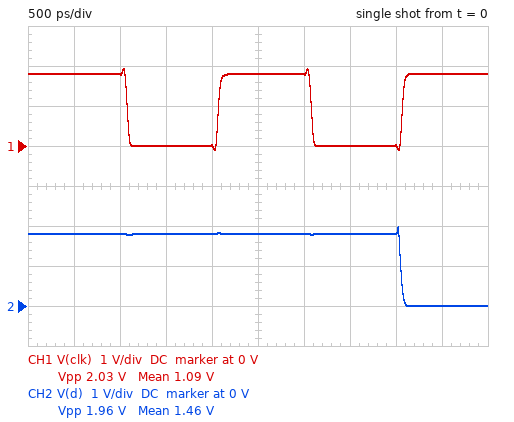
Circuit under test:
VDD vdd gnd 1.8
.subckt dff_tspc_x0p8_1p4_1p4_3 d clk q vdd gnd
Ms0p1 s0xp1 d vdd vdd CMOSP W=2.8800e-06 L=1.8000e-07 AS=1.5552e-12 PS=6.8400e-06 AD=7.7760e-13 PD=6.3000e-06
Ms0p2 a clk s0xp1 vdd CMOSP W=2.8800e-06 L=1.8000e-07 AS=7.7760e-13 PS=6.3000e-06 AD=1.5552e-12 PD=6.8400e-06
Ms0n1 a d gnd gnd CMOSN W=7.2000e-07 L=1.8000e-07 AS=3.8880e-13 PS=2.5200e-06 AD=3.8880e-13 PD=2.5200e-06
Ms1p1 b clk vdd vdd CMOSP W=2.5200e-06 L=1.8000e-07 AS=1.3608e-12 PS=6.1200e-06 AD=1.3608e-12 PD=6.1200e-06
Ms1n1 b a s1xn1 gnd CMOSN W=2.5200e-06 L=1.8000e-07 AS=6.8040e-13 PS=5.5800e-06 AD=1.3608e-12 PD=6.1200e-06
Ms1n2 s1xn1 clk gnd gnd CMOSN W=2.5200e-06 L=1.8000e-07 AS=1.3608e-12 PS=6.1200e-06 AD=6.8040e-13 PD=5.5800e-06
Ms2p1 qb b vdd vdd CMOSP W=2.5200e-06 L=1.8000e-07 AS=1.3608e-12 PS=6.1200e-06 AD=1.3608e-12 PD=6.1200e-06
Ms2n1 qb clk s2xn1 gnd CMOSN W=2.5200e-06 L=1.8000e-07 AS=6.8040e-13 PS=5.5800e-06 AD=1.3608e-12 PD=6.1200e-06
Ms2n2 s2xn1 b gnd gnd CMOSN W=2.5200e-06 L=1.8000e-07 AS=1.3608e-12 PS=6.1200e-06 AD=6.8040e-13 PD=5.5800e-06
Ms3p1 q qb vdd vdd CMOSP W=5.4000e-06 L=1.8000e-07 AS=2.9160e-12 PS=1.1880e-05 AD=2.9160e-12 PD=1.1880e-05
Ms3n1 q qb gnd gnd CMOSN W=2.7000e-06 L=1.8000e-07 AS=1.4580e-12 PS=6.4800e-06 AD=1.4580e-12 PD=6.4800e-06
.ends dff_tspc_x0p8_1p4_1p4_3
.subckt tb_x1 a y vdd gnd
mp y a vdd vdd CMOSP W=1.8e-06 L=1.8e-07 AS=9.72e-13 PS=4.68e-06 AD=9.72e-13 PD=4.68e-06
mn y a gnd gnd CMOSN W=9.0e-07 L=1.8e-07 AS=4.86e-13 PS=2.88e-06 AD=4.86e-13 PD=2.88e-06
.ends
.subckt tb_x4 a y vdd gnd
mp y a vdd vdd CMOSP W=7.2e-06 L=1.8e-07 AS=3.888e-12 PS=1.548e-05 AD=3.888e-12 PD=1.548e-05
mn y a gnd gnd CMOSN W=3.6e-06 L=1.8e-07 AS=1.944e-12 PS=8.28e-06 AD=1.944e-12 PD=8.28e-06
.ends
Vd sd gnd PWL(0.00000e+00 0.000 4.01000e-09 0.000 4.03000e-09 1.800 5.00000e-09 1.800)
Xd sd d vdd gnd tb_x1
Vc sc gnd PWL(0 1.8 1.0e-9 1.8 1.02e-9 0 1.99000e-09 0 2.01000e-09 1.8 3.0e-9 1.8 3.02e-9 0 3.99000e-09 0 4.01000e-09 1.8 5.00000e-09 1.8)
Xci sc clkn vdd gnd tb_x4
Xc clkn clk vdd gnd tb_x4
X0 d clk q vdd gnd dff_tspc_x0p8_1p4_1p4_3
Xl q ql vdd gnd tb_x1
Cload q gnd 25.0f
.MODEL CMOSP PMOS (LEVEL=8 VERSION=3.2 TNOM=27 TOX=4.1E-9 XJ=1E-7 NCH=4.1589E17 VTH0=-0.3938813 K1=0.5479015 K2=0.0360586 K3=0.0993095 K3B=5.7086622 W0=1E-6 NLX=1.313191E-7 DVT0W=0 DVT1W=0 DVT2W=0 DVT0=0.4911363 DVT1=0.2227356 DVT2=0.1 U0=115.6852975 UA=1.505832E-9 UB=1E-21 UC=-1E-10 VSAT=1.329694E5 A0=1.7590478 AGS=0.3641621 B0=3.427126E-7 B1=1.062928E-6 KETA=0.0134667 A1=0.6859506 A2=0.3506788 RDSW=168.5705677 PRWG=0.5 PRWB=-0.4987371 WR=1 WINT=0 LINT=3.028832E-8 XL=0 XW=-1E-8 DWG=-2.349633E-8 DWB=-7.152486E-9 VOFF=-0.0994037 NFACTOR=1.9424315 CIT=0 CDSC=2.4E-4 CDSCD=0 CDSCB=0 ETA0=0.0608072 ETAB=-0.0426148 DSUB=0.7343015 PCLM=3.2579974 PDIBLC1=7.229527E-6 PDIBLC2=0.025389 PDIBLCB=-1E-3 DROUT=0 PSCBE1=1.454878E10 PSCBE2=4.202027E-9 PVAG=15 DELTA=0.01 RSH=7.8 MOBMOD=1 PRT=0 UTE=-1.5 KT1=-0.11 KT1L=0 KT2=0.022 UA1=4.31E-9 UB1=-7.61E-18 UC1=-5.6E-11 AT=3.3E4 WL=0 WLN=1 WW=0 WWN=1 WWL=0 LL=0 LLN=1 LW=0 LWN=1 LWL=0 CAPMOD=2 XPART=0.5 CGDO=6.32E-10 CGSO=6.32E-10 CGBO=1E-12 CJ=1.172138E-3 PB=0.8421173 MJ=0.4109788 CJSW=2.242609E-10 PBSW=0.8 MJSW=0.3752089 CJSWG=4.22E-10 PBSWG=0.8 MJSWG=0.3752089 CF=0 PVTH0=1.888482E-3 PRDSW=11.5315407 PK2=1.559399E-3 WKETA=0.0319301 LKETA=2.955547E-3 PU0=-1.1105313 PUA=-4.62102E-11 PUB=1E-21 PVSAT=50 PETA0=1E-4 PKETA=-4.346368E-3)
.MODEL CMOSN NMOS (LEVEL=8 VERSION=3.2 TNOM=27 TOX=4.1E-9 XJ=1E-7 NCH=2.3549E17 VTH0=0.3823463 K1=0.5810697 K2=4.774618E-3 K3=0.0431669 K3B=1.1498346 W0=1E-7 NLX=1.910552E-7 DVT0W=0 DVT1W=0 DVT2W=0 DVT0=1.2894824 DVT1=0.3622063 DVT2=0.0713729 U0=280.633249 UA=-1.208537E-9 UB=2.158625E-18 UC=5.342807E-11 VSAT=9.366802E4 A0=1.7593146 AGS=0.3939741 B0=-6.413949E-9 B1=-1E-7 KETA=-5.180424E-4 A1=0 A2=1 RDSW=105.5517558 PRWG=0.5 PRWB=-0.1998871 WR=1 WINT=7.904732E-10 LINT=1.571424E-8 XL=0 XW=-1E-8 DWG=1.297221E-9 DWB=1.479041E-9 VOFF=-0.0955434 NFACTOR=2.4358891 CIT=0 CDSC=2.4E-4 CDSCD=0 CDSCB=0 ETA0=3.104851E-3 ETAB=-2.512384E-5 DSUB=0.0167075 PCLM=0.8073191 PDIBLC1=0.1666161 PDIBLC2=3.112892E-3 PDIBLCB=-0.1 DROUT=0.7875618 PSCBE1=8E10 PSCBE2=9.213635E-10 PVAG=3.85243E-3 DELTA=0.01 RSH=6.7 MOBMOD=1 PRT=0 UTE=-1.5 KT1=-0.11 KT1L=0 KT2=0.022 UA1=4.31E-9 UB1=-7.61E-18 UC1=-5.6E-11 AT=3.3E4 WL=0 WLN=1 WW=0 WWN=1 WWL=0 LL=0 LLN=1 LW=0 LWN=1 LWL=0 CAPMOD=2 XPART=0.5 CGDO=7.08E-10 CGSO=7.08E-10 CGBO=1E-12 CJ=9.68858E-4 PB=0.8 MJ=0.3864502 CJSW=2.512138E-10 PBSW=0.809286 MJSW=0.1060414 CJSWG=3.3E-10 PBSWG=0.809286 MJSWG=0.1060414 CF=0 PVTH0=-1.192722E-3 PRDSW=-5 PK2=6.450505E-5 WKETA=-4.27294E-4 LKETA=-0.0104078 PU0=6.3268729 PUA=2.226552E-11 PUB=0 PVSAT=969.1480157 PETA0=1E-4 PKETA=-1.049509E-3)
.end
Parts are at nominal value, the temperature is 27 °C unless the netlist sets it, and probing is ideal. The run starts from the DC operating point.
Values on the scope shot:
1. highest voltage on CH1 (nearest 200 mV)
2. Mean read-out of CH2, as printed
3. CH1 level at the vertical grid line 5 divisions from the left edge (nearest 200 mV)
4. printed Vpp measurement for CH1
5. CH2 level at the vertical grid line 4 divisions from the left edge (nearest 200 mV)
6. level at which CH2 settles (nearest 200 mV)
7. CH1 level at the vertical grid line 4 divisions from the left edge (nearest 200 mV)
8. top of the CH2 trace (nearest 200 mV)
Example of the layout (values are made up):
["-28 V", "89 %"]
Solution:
["2.0 V", "1.46 V", "1.8 V", "2.03 V", "1.8 V", "0 V", "0 V", "2.0 V"]
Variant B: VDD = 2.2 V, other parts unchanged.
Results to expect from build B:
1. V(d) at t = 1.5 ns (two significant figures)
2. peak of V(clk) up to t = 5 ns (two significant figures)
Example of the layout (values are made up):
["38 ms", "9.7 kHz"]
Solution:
["2.2 V", "2.3 V"]
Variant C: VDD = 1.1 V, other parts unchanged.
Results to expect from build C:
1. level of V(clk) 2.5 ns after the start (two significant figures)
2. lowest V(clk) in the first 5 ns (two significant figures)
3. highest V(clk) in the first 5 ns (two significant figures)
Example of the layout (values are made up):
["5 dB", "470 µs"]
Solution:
["1.1 V", "-180 mV", "1.2 V"]
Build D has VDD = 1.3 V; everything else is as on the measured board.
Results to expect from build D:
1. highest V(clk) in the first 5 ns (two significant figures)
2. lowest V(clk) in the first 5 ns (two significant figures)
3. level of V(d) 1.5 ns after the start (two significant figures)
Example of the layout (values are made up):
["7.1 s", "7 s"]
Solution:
["1.4 V", "-160 mV", "1.3 V"]
